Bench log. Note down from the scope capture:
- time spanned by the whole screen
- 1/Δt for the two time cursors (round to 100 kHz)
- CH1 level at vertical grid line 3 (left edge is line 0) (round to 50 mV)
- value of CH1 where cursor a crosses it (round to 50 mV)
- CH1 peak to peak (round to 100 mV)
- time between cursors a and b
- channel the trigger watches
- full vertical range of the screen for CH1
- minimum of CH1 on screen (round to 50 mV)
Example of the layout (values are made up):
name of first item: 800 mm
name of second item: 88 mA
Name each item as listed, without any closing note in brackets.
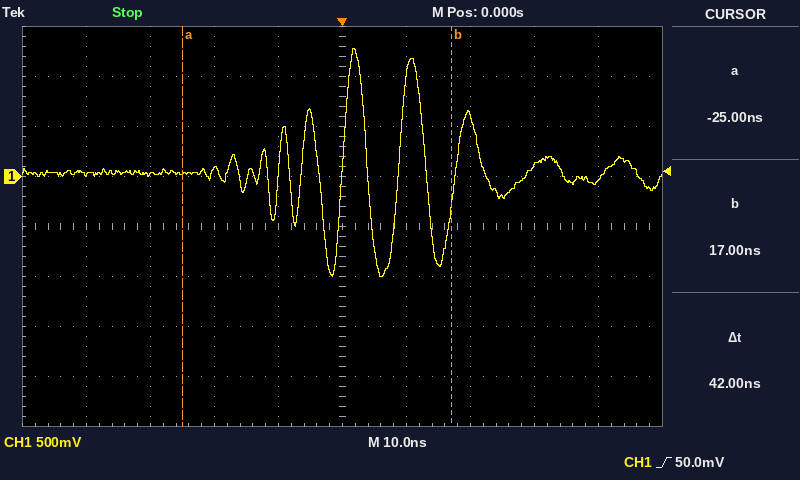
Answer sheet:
time spanned by the whole screen: 100 ns
1/Δt for the two time cursors: 23.8 MHz
CH1 level at vertical grid line 3 (left edge is line 0): 50 mV
value of CH1 where cursor a crosses it: 50 mV
CH1 peak to peak: 2.30 V
time between cursors a and b: 42 ns
channel the trigger watches: CH1
full vertical range of the screen for CH1: 4 V
minimum of CH1 on screen: -1.00 V
